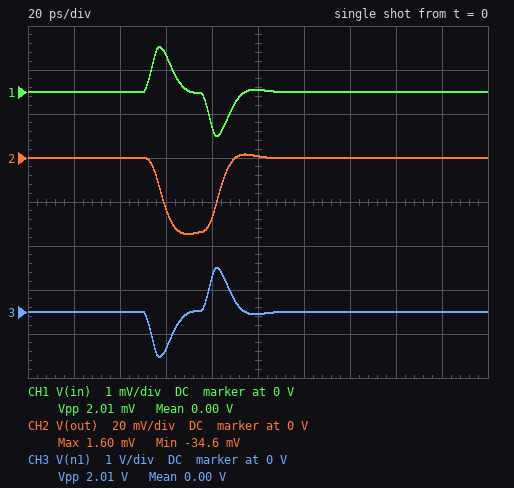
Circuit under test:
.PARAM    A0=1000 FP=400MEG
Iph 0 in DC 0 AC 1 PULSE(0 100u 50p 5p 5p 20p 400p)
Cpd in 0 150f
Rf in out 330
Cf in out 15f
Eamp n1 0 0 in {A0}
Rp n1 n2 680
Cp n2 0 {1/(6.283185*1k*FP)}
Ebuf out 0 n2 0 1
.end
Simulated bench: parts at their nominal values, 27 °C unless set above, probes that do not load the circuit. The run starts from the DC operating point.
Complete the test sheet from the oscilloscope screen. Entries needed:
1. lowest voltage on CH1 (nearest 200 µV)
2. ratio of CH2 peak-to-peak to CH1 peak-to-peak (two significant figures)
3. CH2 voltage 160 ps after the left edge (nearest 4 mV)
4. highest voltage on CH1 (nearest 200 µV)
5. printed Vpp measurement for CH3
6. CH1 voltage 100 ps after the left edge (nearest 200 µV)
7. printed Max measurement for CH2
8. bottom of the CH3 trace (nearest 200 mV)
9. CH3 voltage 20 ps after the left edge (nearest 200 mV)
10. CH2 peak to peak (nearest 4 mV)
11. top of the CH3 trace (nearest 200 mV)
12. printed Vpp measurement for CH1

-1.0 mV
18
0 V
1.0 mV
2.01 V
0 V
1.60 mV
-1.0 V
0 V
36 mV
1.0 V
2.01 mV
